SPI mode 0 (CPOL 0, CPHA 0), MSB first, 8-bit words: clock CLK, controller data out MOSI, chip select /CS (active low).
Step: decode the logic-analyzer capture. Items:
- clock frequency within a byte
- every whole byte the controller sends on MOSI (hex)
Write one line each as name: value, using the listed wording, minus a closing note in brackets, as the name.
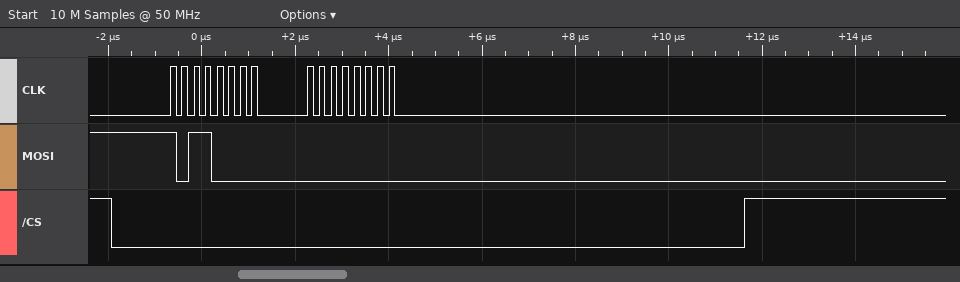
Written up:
clock frequency within a byte: 4 MHz
every whole byte the controller sends on MOSI: B0 00
